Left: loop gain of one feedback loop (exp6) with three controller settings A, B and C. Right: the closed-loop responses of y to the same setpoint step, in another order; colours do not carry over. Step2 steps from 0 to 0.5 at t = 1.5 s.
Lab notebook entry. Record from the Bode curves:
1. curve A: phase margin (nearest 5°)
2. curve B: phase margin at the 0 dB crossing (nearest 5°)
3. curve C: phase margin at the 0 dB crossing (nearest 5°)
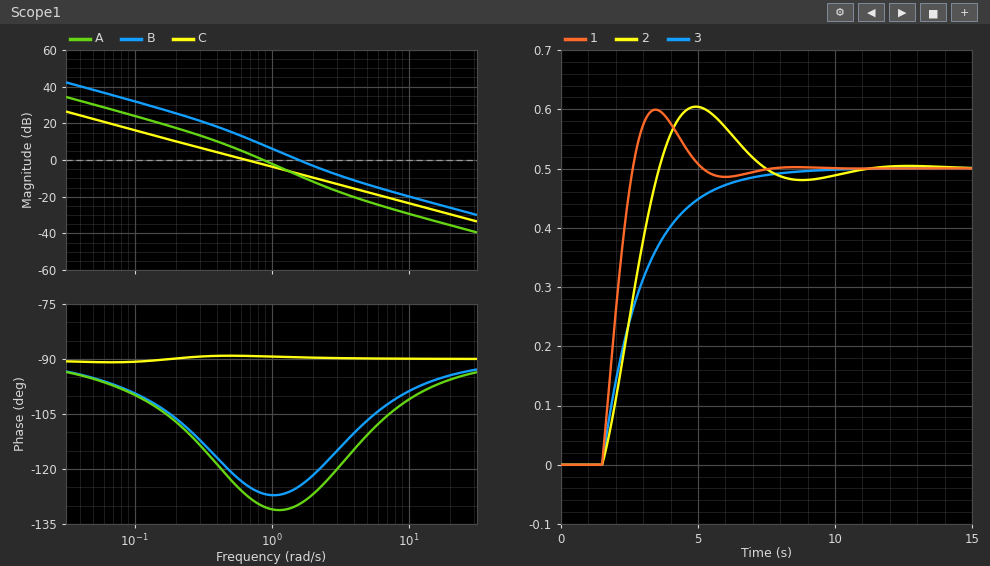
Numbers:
50°
55°
90°
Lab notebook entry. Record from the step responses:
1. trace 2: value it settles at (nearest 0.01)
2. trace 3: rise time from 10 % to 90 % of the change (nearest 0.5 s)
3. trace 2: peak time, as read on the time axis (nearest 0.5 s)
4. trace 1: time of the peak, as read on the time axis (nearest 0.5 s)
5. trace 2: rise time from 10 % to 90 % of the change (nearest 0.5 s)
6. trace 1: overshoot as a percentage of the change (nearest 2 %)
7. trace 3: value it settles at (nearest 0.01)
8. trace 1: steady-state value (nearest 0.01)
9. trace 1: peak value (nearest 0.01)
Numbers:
0.50
3.5 s
5.0 s
3.5 s
1.5 s
20 %
0.50
0.50
0.60
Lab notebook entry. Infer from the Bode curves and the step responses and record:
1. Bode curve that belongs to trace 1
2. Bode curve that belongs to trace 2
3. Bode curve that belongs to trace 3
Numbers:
B
A
C
